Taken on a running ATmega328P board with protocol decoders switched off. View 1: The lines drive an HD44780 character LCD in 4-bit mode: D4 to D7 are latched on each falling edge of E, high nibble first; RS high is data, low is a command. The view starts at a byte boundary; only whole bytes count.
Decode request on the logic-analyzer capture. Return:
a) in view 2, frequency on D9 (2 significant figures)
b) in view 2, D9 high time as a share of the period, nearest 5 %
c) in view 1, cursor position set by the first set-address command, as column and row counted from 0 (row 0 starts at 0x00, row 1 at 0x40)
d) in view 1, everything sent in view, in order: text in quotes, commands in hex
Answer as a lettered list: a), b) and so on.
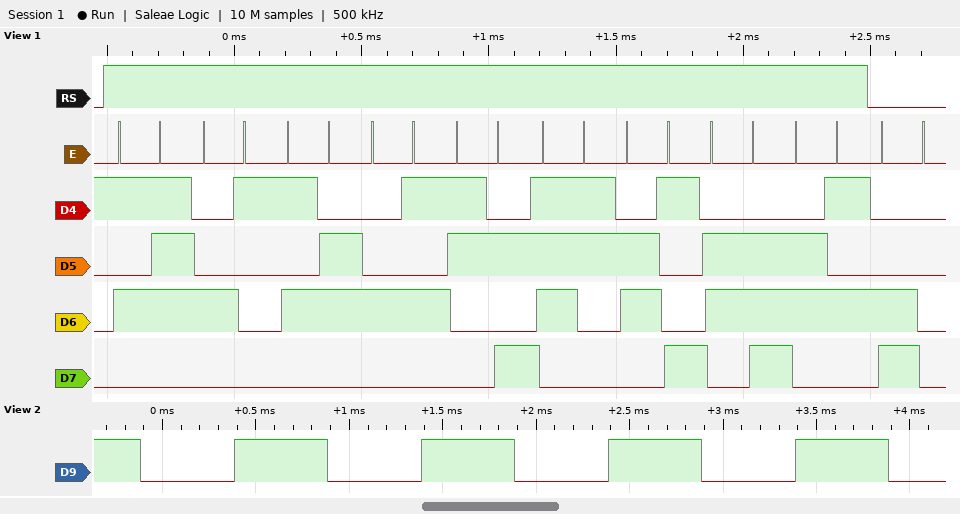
a) 1.0 kHz
b) 50 %
c) column 0, row 1
d) "WAVE:sine" 0xC0
